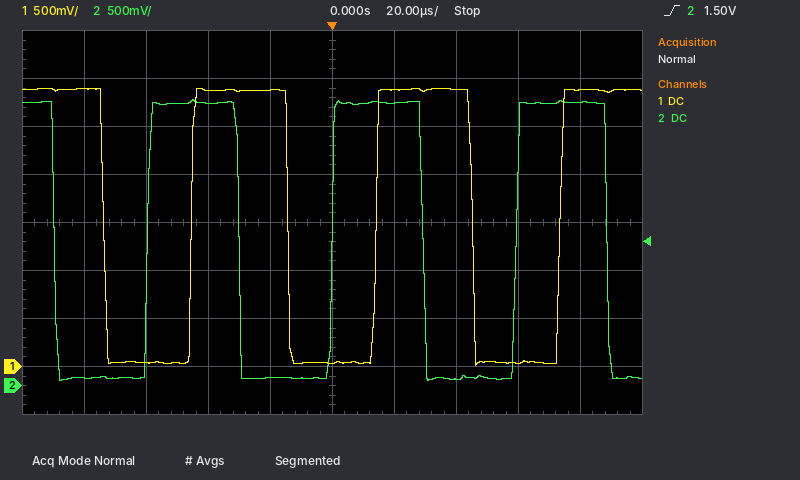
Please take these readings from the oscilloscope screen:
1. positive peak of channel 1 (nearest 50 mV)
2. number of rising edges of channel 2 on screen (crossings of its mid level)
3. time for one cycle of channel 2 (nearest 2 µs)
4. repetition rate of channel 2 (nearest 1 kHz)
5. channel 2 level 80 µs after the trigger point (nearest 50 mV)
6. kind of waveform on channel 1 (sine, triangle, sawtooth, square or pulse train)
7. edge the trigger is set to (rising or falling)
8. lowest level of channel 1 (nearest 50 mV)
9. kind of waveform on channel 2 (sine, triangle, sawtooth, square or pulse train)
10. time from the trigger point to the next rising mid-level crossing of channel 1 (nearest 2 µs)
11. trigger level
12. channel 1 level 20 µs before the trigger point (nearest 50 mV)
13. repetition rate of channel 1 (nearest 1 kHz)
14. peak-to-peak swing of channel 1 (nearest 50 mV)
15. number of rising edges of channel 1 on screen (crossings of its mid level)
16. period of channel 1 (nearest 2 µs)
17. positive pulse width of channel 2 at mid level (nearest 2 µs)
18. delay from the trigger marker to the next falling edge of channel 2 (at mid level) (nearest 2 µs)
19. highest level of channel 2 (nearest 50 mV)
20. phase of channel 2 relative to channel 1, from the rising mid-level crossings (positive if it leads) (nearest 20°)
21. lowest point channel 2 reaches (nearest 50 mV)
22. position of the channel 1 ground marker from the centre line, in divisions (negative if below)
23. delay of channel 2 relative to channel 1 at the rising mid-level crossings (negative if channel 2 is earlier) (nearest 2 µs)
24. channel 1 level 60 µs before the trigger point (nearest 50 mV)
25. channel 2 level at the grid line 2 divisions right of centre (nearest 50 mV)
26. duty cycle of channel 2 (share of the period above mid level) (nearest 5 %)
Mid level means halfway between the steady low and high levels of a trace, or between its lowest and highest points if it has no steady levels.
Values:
2.90 V
3
60 µs
17 kHz
2.95 V
square
rising
0 mV
square
14 µs
1.50 V
2.90 V
17 kHz
2.90 V
3
60 µs
30 µs
30 µs
3.00 V
+80°
50 mV
-3.0 div
-14 µs
50 mV
50 mV
50 %
